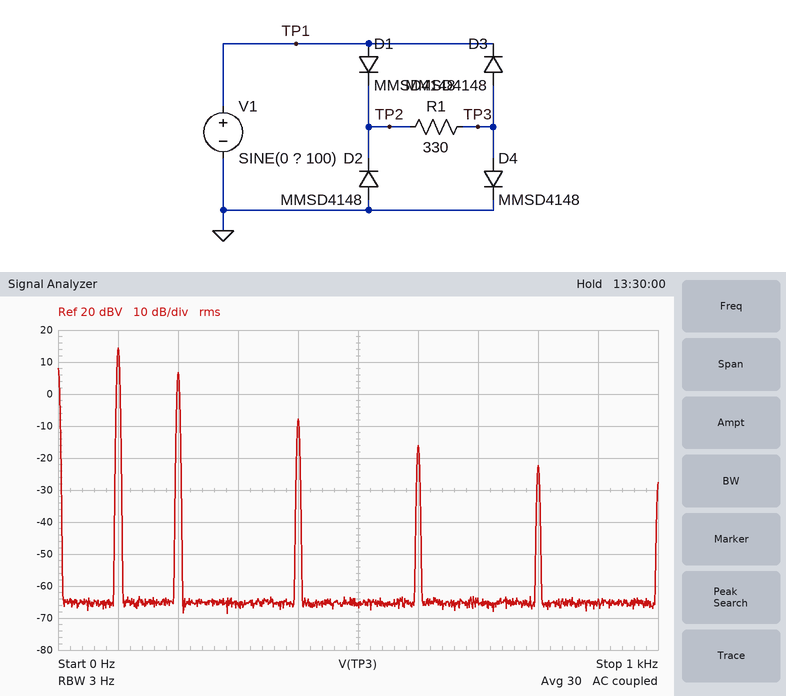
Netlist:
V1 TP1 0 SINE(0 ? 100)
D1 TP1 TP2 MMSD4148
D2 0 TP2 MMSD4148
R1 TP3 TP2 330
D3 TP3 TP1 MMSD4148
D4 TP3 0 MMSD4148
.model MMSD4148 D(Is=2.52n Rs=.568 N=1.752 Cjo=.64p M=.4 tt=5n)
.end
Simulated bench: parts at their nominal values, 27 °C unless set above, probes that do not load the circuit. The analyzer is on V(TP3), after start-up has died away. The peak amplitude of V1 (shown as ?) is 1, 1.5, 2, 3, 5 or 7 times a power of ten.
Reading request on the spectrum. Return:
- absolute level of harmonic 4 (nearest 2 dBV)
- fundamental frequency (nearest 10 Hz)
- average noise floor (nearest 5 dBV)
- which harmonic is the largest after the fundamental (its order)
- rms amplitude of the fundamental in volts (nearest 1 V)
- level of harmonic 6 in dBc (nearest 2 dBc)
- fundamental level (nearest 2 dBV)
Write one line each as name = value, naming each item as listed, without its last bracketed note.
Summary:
absolute level of harmonic 4 = -8 dBV
fundamental frequency = 100 Hz
average noise floor = -65 dBV
which harmonic is the largest after the fundamental = 2
rms amplitude of the fundamental in volts = 5 V
level of harmonic 6 in dBc = -30 dBc
fundamental level = 14 dBV
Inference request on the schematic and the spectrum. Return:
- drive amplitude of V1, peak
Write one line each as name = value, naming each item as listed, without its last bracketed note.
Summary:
drive amplitude of V1, peak = 15 V
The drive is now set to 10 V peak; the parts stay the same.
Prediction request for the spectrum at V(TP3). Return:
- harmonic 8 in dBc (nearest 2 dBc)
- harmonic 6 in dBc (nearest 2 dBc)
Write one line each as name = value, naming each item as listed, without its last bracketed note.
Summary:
harmonic 8 in dBc = -40 dBc
harmonic 6 in dBc = -32 dBc
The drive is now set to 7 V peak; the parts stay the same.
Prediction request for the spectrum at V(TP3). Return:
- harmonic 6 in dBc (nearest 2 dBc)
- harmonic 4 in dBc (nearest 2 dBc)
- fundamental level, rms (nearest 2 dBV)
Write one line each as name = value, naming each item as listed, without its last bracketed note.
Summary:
harmonic 6 in dBc = -36 dBc
harmonic 4 in dBc = -24 dBc
fundamental level, rms = 8 dBV
